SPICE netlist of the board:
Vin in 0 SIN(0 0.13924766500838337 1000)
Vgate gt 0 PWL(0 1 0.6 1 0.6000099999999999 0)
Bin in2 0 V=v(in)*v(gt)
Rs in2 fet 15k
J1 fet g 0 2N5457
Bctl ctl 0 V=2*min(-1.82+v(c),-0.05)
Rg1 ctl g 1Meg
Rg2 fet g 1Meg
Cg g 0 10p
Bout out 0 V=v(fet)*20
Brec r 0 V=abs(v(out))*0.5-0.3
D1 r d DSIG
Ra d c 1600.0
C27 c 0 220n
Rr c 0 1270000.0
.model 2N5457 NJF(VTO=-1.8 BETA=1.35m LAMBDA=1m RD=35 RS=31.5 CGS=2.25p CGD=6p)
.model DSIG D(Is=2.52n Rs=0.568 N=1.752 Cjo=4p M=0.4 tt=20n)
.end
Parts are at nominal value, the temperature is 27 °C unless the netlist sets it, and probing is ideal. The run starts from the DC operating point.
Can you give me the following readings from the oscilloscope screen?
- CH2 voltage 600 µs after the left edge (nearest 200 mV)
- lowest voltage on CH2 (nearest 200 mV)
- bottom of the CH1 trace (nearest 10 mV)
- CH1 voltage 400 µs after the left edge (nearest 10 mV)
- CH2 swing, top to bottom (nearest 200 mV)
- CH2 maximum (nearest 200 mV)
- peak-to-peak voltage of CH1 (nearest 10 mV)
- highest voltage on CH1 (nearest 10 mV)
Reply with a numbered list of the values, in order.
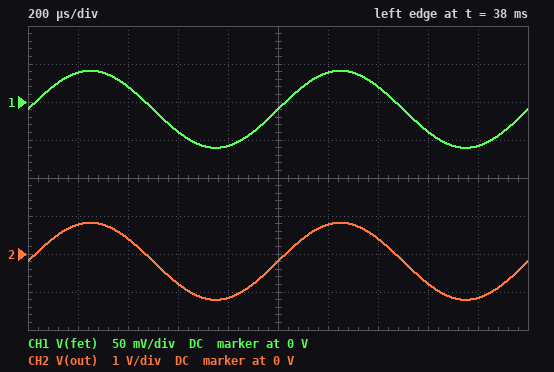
1. -800 mV
2. -1.2 V
3. -60 mV
4. 20 mV
5. 2.0 V
6. 800 mV
7. 100 mV
8. 40 mV
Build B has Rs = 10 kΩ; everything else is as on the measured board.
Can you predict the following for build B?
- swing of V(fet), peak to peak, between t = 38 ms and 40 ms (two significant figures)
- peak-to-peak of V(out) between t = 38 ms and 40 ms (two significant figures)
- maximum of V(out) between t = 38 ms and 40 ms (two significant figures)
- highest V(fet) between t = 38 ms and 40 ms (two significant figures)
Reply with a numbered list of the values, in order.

1. 110 mV
2. 2.2 V
3. 970 mV
4. 49 mV
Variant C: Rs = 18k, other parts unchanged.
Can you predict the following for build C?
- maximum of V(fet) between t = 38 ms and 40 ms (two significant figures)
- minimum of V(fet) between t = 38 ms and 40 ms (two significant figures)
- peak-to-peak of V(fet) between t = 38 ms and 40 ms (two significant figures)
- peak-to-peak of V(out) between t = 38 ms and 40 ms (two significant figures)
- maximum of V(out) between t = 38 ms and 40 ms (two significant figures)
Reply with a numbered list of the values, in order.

1. 37 mV
2. -59 mV
3. 97 mV
4. 1.9 V
5. 750 mV
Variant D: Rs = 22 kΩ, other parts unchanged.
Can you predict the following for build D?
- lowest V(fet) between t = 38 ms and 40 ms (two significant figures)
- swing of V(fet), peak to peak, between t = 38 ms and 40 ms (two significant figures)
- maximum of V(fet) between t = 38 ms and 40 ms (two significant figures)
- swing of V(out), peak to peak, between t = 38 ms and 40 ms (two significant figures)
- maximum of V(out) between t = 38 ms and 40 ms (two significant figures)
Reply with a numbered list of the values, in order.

1. -58 mV
2. 91 mV
3. 33 mV
4. 1.8 V
5. 660 mV
